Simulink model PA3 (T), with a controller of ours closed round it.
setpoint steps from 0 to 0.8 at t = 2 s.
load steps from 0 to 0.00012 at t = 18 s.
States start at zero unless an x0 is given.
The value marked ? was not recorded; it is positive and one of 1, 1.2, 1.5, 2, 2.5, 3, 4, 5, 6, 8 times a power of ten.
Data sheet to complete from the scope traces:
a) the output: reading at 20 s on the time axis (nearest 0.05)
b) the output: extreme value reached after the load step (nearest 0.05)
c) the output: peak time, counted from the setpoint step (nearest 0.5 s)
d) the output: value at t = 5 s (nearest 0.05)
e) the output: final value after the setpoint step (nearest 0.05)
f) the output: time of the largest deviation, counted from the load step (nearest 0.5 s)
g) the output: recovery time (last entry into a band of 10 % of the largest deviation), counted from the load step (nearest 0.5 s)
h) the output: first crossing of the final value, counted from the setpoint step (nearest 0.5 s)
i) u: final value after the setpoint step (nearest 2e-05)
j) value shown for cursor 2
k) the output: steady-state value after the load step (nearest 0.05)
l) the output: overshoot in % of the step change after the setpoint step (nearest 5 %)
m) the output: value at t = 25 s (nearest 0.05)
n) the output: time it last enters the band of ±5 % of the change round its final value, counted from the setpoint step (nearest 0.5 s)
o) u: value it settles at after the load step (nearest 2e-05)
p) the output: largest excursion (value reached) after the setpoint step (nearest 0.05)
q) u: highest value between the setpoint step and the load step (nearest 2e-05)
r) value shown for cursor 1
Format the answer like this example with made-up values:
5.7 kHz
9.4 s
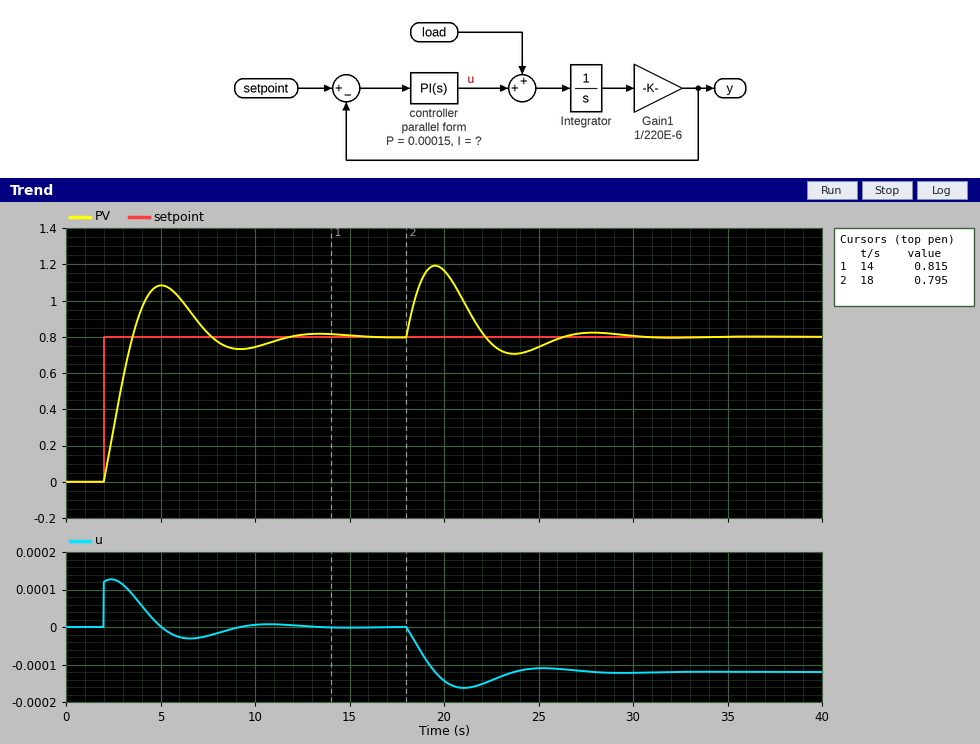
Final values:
1.15
1.20
3.0 s
1.10
0.80
1.5 s
7.5 s
1.5 s
0.00000
0.795
0.80
35 %
0.75
8.5 s
-0.00012
1.10
0.00012
0.815
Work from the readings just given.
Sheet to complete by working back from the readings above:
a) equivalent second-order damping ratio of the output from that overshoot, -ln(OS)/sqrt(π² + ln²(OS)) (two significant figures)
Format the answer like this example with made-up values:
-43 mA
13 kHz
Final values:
0.32
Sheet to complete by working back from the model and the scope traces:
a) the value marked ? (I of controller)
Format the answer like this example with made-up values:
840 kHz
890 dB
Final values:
0.00015
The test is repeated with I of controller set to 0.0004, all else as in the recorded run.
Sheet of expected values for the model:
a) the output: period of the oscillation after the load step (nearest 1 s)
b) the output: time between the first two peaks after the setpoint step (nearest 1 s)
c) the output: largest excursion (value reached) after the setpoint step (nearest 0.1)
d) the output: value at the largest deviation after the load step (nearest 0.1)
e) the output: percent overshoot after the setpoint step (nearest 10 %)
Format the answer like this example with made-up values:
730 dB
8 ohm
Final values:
5 s
5 s
1.2
1.1
50 %
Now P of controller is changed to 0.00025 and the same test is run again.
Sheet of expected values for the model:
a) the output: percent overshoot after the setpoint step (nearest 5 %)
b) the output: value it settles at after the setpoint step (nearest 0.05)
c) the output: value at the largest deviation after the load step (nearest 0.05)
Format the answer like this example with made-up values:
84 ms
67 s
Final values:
20 %
0.80
1.10
